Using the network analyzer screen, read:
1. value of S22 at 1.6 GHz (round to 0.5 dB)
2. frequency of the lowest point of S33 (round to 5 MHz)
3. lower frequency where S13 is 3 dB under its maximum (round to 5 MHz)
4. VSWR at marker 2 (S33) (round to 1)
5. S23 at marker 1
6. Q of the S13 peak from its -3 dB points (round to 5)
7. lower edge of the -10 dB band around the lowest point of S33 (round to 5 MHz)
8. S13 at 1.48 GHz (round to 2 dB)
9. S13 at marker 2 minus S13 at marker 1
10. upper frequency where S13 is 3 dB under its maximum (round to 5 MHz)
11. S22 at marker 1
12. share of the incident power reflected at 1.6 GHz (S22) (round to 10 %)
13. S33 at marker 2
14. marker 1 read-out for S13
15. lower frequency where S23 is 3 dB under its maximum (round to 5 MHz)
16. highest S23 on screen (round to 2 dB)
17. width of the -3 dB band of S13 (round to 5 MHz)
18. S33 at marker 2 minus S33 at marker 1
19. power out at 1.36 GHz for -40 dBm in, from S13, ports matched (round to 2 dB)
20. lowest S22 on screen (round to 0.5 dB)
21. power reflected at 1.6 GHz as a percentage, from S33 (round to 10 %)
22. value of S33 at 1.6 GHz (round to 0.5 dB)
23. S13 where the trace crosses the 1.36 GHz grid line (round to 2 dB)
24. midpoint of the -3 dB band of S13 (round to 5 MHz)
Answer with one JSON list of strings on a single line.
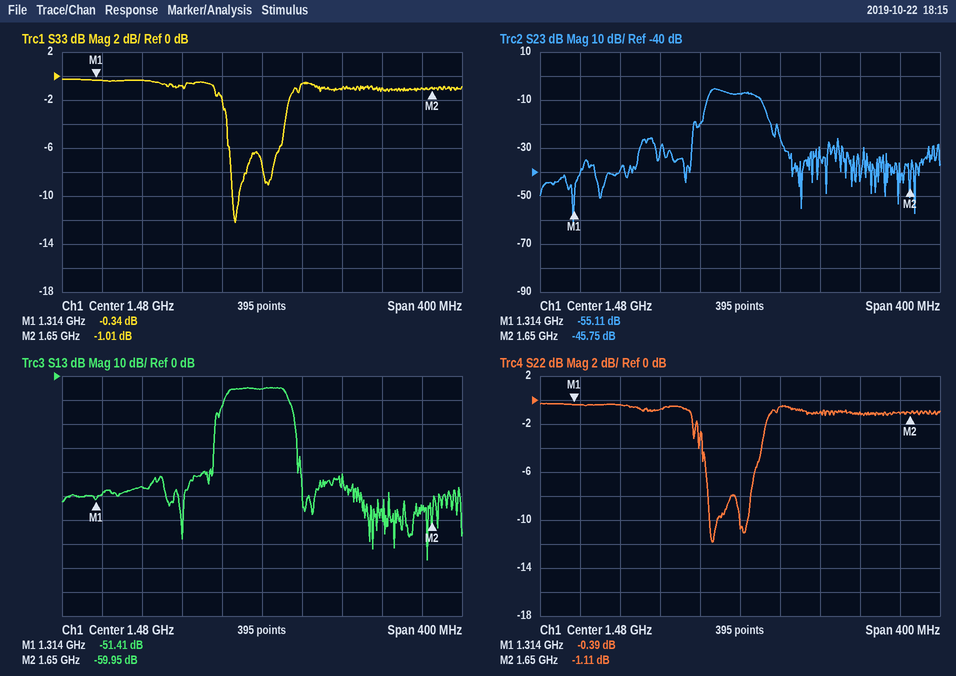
["-1.0 dB", "1.455 GHz", "1.445 GHz", "17", "-55.11 dB", "25", "1.450 GHz", "-6 dB", "-8.54 dB", "1.505 GHz", "-0.39 dB", "80 %", "-1.01 dB", "-51.41 dB", "1.450 GHz", "-6 dB", "60 MHz", "-0.67 dB", "-86 dBm", "-12.0 dB", "80 %", "-1.0 dB", "-46 dB", "1.475 GHz"]
